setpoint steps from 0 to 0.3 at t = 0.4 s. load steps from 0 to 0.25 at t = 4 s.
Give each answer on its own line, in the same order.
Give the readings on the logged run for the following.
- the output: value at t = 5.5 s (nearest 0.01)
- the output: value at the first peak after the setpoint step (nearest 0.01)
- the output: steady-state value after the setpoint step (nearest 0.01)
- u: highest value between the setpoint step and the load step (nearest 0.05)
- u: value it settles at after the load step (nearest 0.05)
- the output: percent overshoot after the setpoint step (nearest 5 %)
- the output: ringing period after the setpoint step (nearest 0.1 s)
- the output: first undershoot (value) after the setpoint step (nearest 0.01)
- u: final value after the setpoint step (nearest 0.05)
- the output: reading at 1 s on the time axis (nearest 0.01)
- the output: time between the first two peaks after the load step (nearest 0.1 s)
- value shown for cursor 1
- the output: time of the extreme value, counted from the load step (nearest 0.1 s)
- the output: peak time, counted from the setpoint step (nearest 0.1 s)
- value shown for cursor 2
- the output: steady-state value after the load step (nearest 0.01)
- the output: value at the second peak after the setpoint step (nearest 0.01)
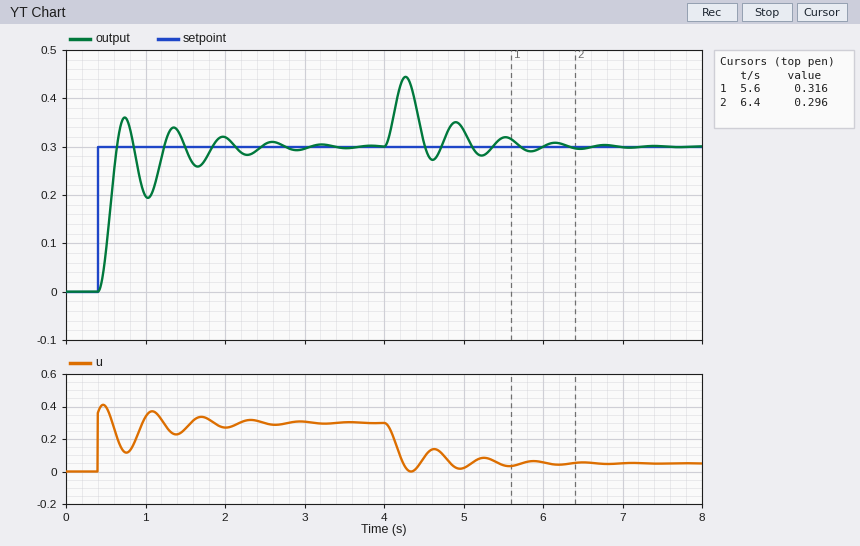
0.32
0.36
0.30
0.40
0.05
20 %
0.6 s
0.19
0.30
0.20
0.6 s
0.316
0.3 s
0.3 s
0.296
0.30
0.34
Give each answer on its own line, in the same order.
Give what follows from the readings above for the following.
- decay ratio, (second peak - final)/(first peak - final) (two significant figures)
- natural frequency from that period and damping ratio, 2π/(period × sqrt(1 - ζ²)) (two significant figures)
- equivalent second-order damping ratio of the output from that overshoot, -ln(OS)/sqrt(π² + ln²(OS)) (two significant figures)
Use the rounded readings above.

0.67
12 rad/s
0.46
